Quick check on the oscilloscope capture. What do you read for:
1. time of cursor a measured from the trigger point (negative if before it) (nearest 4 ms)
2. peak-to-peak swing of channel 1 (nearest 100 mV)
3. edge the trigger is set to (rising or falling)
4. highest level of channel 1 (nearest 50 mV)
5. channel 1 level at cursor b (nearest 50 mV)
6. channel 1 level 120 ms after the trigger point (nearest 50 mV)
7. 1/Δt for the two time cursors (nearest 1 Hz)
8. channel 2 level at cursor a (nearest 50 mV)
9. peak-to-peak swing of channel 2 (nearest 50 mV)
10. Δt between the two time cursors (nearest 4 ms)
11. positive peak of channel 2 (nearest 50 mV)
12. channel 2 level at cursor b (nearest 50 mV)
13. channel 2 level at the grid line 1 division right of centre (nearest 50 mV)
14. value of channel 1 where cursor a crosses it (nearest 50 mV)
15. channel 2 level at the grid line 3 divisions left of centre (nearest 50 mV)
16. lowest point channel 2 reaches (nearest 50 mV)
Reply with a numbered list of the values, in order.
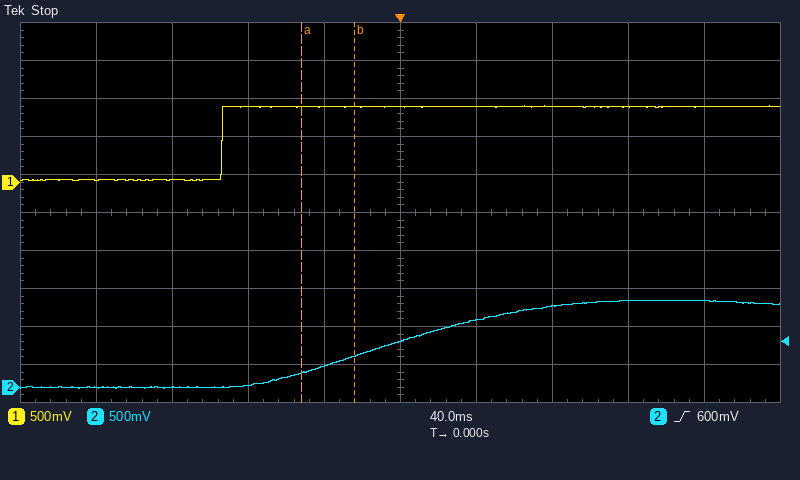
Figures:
1. -52 ms
2. 1.00 V
3. rising
4. 1.00 V
5. 1.00 V
6. 1.00 V
7. 36 Hz
8. 200 mV
9. 1.15 V
10. 28 ms
11. 1.15 V
12. 400 mV
13. 900 mV
14. 1.00 V
15. 0 mV
16. 0 mV
